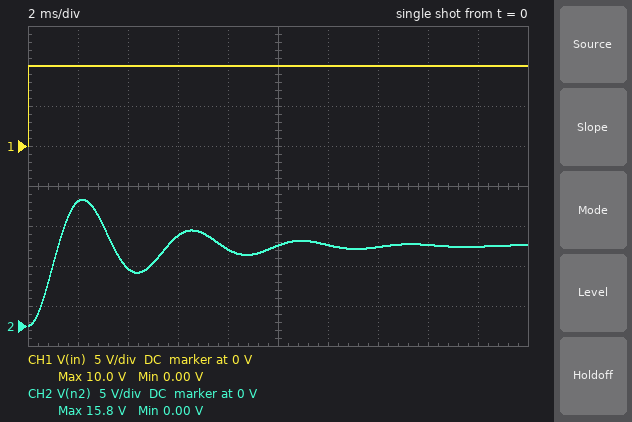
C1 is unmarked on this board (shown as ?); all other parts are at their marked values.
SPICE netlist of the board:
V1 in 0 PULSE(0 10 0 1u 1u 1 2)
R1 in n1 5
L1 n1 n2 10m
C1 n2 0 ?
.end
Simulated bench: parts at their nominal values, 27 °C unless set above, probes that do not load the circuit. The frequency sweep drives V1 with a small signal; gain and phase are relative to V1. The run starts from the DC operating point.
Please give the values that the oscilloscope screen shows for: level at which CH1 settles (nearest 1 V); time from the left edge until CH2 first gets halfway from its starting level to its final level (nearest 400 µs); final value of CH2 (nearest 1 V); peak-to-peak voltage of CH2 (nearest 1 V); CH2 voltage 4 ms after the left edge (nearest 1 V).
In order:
10 V
800 µs
10 V
16 V
7 V
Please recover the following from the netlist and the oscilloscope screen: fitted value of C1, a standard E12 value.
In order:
47 µF
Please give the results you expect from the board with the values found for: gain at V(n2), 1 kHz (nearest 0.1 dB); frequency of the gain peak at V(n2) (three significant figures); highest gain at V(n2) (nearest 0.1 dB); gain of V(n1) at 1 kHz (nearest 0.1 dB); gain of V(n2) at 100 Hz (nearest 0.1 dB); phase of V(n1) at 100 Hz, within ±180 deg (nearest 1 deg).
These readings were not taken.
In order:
-24.9 dB
225 Hz
9.4 dB
0 dB
1.6 dB
-10 deg
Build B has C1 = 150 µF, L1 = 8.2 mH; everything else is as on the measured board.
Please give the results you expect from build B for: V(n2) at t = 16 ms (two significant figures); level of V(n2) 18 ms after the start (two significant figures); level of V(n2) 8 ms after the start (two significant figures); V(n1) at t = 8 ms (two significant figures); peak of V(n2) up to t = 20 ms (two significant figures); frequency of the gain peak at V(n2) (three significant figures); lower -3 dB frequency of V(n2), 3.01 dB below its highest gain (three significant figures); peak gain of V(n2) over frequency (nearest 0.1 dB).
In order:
9.9 V
10 V
9.1 V
9.7 V
13 V
126 Hz
52.7 Hz
3.9 dB
